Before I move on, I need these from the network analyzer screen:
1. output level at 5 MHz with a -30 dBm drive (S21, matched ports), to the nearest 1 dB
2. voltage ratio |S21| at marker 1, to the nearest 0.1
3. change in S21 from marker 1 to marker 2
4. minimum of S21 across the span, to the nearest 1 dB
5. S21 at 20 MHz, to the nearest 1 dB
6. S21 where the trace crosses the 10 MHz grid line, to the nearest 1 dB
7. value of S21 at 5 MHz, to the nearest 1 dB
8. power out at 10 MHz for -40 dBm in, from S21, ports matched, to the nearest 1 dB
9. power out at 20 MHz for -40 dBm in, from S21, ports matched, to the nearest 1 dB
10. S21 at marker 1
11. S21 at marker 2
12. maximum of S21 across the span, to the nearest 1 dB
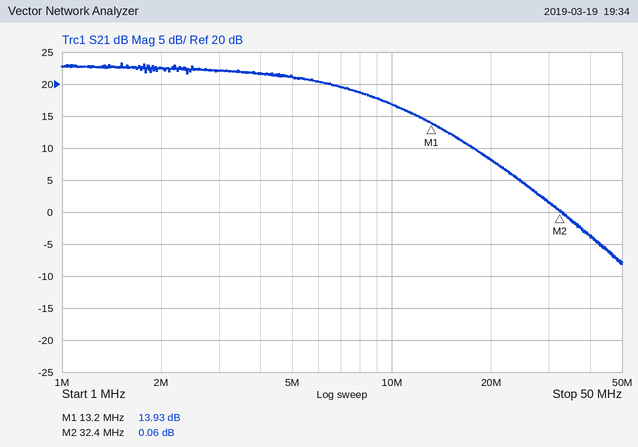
-9 dBm
5.0
-13.87 dB
-8 dB
8 dB
17 dB
21 dB
-23 dBm
-32 dBm
13.93 dB
0.06 dB
23 dB
